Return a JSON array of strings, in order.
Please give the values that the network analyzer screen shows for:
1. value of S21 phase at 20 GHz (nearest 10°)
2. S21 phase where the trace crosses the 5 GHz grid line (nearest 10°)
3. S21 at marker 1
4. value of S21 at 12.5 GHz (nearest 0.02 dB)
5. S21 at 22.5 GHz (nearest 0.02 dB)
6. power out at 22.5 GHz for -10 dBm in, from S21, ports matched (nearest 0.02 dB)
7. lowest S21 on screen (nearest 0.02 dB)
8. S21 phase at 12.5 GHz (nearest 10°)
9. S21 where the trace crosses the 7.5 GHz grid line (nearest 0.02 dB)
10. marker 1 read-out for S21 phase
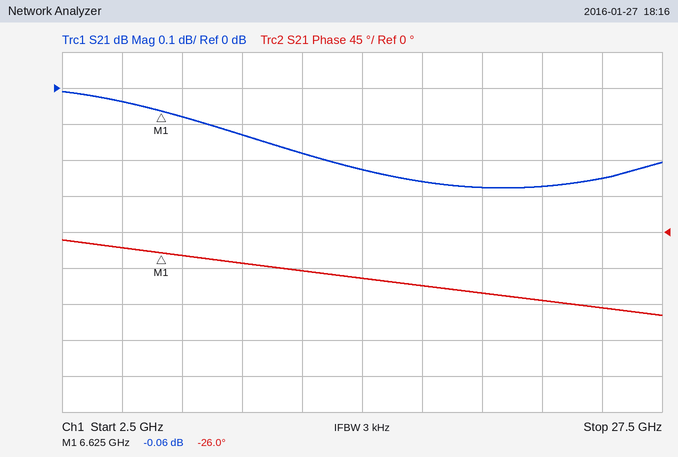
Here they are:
["-80°", "-20°", "-0.06 dB", "-0.18 dB", "-0.28 dB", "-10.28 dBm", "-0.28 dB", "-50°", "-0.08 dB", "-26.0°"]
